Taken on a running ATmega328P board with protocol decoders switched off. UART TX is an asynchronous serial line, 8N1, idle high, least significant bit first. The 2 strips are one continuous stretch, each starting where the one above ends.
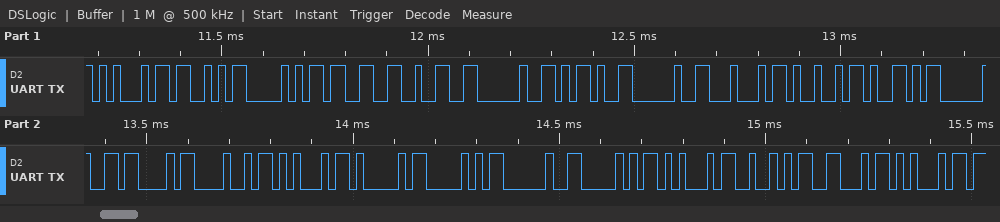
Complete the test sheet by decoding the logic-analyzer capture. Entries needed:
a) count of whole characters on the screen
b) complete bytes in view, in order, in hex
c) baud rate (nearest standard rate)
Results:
23
45 53 50 33 32 20 2D 20 44 49 59 20 43 48 45 41 50 20 50 45 52 46 45
57600 baud
